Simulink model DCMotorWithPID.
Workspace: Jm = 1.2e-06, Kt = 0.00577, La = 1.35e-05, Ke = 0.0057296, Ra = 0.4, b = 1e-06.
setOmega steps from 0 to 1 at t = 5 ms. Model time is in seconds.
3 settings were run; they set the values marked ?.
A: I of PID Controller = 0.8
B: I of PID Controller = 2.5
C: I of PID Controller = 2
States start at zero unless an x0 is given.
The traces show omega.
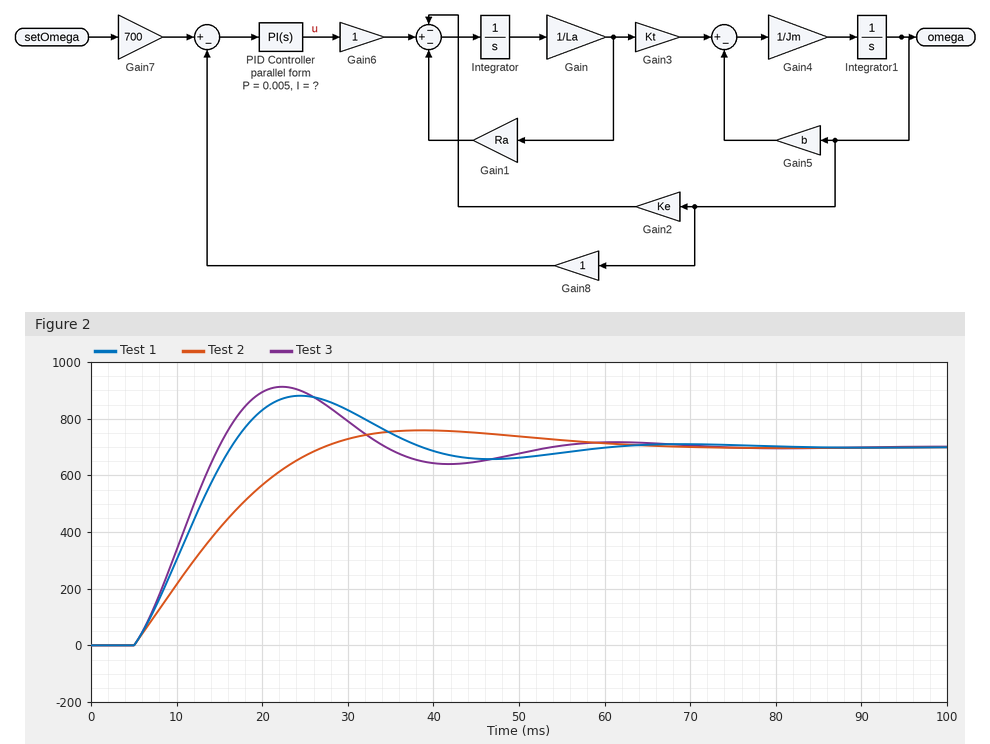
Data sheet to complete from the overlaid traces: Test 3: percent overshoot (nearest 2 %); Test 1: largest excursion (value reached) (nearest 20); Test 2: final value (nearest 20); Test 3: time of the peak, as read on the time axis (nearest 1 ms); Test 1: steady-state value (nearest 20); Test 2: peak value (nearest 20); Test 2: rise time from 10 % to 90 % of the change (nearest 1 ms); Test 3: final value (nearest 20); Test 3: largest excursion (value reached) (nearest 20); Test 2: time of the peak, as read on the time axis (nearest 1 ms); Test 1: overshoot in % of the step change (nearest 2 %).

30 %
880
700
22 ms
700
760
16 ms
700
920
39 ms
26 %
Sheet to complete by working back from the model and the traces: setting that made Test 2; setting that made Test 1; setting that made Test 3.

A
C
B
